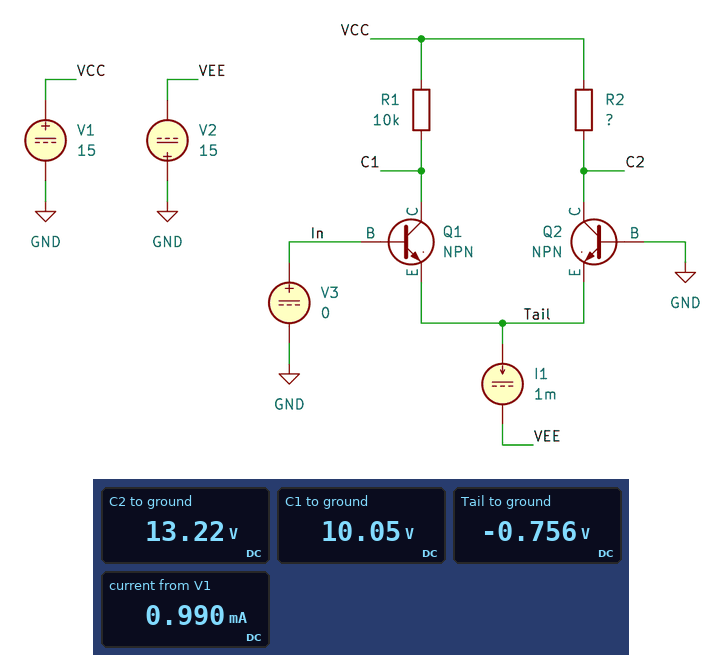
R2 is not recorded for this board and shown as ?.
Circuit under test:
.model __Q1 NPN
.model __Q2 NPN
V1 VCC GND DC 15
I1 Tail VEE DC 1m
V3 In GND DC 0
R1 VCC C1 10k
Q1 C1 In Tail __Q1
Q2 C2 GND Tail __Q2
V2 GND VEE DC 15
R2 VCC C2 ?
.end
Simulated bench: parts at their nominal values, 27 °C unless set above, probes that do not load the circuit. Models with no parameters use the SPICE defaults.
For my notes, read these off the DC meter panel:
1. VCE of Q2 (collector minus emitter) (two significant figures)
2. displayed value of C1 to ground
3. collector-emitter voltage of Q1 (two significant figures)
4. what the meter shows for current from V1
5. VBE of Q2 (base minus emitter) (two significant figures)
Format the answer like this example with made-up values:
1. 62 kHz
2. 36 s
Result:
1. 14 V
2. 10.05 V
3. 11 V
4. 0.990 mA
5. 760 mV
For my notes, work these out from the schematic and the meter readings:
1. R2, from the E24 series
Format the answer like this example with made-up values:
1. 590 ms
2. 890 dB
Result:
1. 3.6 kΩ
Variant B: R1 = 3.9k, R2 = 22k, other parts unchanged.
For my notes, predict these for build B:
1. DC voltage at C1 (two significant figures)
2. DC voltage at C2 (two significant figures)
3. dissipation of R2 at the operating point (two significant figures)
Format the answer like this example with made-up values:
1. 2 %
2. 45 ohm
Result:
1. 13 V
2. 4.1 V
3. 5.4 mW
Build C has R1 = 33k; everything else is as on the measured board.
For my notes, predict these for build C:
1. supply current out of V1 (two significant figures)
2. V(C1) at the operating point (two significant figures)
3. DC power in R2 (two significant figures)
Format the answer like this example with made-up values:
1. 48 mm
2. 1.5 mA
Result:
1. 980 µA
2. -660 mV
3. 910 µW
